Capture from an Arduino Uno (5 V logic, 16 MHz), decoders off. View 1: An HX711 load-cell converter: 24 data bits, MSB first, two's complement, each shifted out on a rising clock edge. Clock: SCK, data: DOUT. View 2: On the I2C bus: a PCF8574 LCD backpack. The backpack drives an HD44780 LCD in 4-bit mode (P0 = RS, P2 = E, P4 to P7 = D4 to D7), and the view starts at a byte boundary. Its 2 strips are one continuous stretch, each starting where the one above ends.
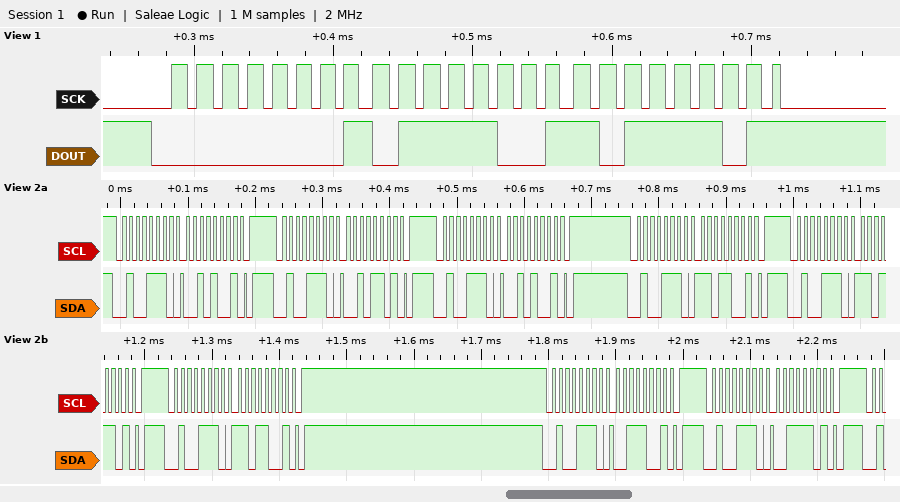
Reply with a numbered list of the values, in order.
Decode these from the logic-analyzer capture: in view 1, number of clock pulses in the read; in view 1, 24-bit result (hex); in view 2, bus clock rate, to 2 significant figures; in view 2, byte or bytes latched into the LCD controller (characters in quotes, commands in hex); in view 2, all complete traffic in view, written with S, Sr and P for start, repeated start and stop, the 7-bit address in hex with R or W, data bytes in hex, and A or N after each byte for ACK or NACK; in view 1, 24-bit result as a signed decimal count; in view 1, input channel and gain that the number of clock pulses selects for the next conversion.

1. 25
2. 0x0179BD
3. 100 kHz
4. '-'
5. S 27W A 29 A P S 27W A 2D A P S 27W A 29 A P S 27W A D9 A P S 27W A DD A P S 27W A D9 A P S 27W A 39 A P S 27W A 3D A P
6. 96701
7. channel A, gain 128
